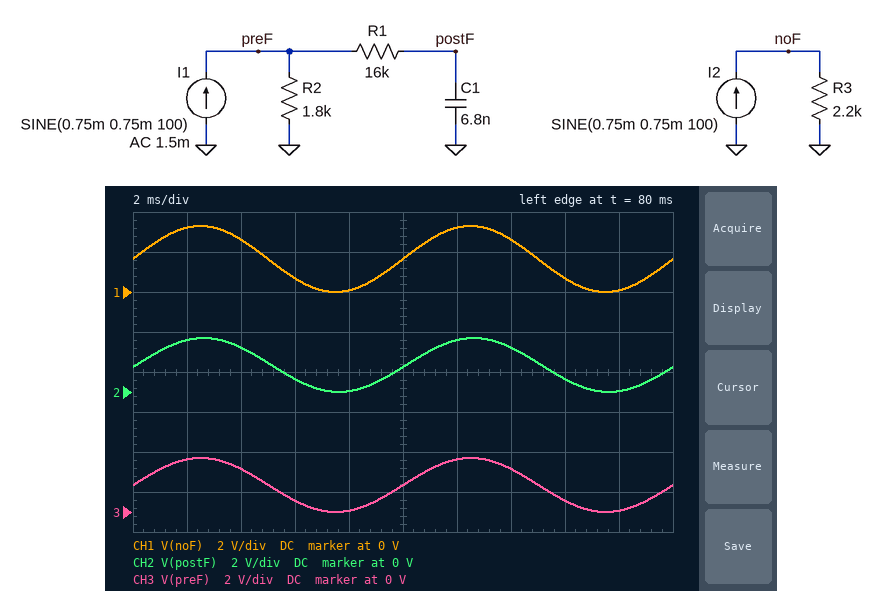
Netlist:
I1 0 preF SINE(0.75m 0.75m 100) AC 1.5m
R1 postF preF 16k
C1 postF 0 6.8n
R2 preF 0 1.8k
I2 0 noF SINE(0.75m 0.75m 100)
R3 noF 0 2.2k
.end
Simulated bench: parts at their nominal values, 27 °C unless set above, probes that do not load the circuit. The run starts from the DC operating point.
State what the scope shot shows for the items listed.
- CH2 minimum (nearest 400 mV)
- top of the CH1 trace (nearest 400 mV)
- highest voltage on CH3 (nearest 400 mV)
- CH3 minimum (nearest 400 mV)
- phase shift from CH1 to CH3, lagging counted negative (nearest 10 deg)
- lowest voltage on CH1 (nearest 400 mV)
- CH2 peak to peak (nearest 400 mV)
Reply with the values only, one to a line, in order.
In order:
0 V
3.2 V
2.8 V
0 V
0 deg
0 V
2.8 V
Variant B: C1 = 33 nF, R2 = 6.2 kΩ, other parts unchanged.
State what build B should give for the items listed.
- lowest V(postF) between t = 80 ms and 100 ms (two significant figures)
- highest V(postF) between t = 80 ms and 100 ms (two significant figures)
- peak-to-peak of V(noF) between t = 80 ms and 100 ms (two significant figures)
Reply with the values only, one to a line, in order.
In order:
430 mV
8.9 V
3.3 V
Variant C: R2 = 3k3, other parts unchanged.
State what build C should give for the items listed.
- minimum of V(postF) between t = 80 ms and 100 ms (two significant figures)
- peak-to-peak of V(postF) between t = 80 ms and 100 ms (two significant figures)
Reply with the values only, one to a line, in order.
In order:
8.4 mV
4.9 V
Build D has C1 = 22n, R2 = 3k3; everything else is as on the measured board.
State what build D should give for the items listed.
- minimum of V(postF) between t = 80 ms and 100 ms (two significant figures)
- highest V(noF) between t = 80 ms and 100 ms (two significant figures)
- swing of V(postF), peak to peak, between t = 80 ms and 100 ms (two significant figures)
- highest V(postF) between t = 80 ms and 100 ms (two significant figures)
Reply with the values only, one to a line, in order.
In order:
84 mV
3.3 V
4.8 V
4.9 V
